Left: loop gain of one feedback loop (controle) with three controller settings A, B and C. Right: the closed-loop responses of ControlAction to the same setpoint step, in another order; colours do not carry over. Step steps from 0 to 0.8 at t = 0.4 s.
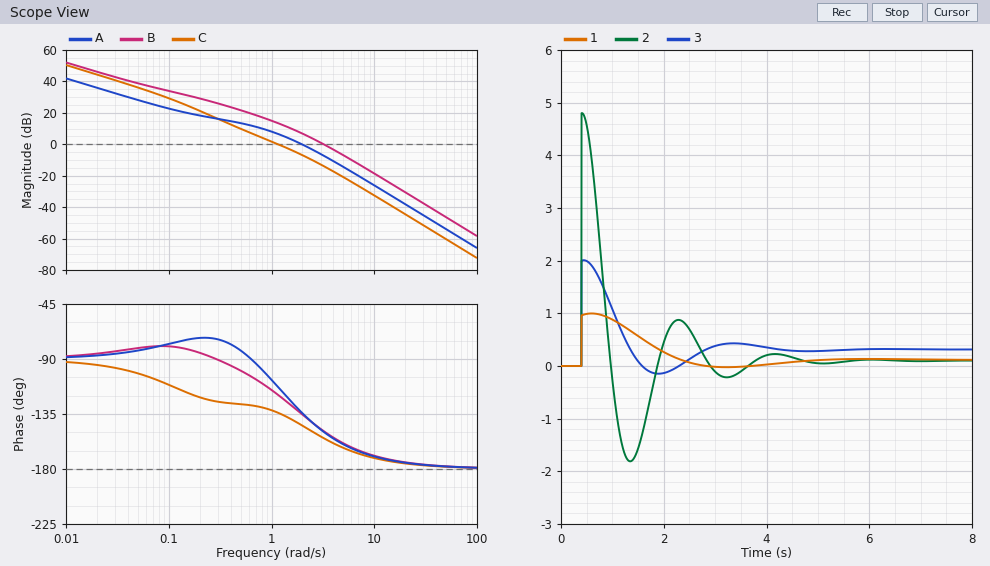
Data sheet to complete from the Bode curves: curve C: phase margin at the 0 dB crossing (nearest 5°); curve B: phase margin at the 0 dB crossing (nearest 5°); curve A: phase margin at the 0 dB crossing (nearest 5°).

45°
30°
45°
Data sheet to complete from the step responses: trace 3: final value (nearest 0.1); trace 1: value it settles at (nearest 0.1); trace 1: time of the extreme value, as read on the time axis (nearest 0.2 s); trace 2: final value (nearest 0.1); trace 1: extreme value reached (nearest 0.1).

0.3
0.1
0.6 s
0.1
1.0
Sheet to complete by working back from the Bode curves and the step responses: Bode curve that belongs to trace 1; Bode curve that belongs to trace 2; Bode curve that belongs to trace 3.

C
B
A
